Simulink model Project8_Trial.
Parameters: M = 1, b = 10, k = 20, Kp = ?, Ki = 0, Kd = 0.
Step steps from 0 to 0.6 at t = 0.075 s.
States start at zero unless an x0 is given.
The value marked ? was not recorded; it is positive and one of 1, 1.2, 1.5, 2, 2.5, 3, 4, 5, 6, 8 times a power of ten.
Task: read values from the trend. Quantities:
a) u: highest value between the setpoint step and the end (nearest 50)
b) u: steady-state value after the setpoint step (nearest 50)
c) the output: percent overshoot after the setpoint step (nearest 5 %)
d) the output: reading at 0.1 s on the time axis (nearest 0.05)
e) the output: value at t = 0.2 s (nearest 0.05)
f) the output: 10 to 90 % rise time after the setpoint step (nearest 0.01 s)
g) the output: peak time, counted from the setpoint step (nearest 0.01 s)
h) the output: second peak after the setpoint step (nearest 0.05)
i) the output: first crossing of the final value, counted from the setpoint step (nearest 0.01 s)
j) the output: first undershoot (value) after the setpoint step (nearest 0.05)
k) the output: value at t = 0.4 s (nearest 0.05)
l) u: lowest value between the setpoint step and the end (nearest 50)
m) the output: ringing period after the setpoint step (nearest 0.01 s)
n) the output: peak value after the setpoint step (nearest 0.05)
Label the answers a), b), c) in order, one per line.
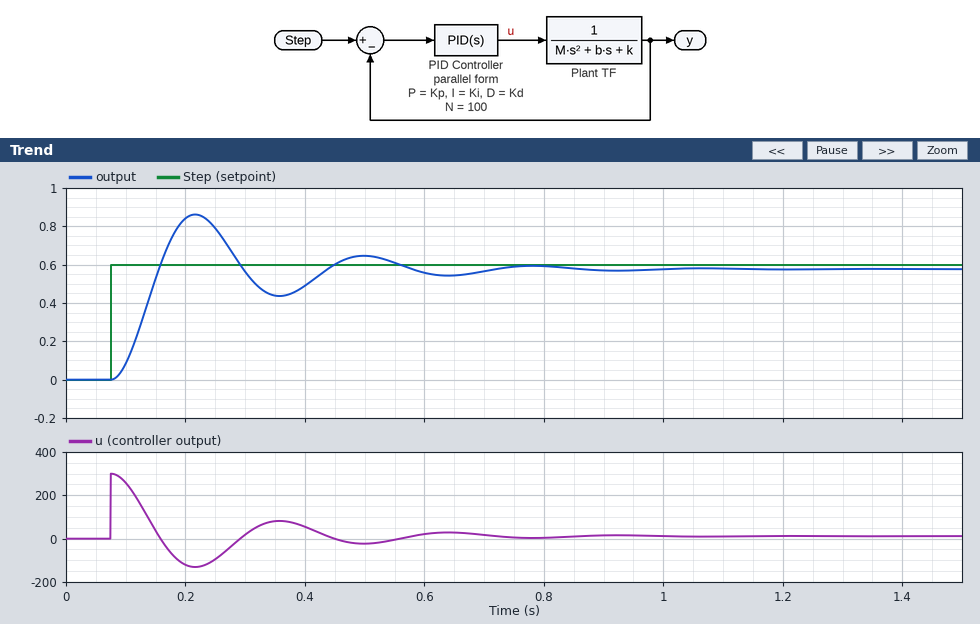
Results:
a) 300
b) 0
c) 50 %
d) 0.10
e) 0.85
f) 0.05 s
g) 0.14 s
h) 0.65
i) 0.08 s
j) 0.45
k) 0.50
l) -150
m) 0.28 s
n) 0.85
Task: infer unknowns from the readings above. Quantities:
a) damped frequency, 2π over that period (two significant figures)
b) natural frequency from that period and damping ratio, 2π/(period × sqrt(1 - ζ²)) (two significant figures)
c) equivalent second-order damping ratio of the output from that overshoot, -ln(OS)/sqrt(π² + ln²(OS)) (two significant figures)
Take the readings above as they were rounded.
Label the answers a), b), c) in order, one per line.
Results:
a) 22 rad/s
b) 23 rad/s
c) 0.22
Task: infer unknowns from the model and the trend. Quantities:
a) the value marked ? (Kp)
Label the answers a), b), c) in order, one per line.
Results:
a) 500
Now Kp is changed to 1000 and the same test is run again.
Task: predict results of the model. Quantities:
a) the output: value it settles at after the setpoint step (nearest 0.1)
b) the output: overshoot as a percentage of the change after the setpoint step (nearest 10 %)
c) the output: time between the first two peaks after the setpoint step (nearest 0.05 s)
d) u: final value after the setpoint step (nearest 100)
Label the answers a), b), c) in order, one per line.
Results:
a) 0.6
b) 60 %
c) 0.20 s
d) 0
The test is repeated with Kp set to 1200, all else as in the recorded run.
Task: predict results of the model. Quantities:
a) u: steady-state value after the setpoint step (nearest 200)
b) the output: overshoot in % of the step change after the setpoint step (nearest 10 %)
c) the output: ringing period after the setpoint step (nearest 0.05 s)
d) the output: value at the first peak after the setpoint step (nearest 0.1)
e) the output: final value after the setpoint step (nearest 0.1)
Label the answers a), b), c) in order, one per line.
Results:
a) 0
b) 60 %
c) 0.20 s
d) 1.0
e) 0.6
